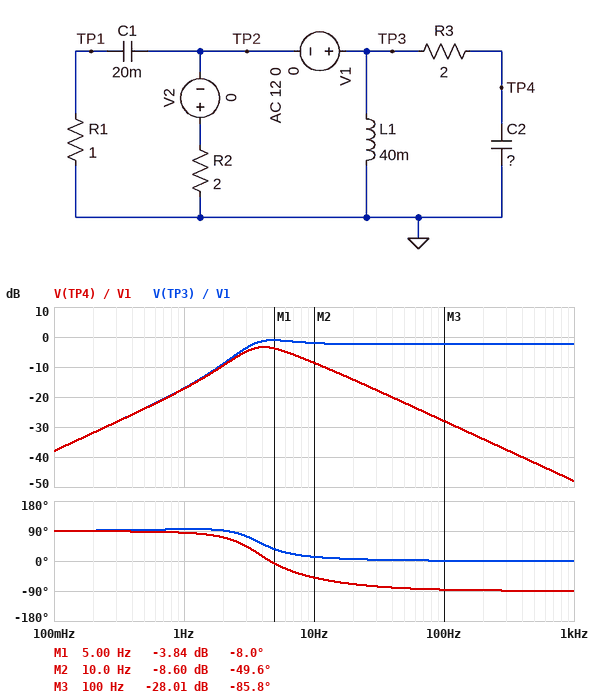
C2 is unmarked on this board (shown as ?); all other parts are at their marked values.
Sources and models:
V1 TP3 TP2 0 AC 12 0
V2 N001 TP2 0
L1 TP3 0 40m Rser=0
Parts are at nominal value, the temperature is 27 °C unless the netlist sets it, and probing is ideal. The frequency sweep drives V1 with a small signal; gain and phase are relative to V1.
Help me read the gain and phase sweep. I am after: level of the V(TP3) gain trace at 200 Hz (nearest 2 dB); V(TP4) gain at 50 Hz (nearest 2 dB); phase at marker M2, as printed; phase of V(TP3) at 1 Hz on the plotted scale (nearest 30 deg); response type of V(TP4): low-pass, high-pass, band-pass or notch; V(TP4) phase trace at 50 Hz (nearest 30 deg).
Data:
-2 dB
-22 dB
-49.6 deg
90 deg
band-pass
-90 deg
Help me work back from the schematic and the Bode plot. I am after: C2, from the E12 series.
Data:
15 mF
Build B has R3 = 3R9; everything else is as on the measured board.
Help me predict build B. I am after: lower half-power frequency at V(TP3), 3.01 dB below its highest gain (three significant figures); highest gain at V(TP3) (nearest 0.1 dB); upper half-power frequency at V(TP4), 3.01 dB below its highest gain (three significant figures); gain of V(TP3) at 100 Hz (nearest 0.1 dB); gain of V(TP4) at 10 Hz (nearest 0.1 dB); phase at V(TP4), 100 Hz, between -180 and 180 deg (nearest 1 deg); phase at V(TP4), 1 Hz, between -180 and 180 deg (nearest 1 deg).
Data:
3.15 Hz
-0.8 dB
7.21 Hz
-1.4 dB
-12.6 dB
-87 deg
75 deg
